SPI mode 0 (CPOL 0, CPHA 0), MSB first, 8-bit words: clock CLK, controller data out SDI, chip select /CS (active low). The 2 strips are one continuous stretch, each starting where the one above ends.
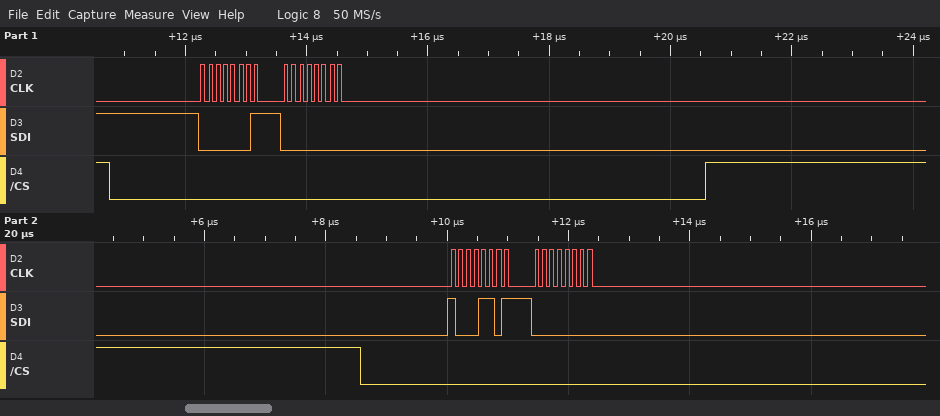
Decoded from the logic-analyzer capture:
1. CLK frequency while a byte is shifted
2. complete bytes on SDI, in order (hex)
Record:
8 MHz
01 00 8D 00
